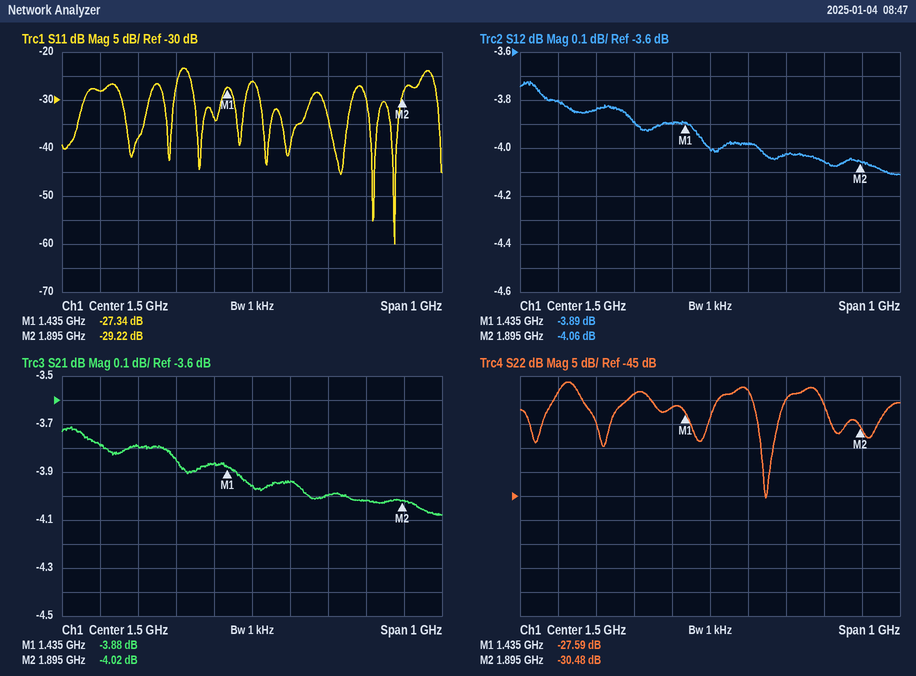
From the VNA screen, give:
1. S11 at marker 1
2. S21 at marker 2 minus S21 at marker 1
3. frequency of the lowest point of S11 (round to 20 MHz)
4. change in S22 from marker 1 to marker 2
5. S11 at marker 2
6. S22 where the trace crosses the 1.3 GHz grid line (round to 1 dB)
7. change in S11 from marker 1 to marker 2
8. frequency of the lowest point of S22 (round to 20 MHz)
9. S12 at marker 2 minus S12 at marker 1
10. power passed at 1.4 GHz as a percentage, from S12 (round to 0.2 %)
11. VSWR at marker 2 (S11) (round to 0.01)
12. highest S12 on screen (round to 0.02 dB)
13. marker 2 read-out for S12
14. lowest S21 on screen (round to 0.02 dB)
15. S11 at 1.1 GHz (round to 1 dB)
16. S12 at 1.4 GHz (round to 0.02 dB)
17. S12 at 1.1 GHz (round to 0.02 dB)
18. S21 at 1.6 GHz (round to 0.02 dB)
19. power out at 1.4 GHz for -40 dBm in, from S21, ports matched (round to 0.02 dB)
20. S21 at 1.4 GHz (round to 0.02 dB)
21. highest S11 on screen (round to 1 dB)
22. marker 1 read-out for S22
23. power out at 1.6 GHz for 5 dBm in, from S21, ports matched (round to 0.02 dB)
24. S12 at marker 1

-27.34 dB
-0.14 dB
1.88 GHz
-2.89 dB
-29.22 dB
-24 dB
-1.88 dB
1.64 GHz
-0.17 dB
40.8 %
1.07
-3.72 dB
-4.06 dB
-4.08 dB
-28 dB
-3.90 dB
-3.80 dB
-3.94 dB
-43.86 dBm
-3.86 dB
-23 dB
-27.59 dB
1.06 dBm
-3.89 dB
